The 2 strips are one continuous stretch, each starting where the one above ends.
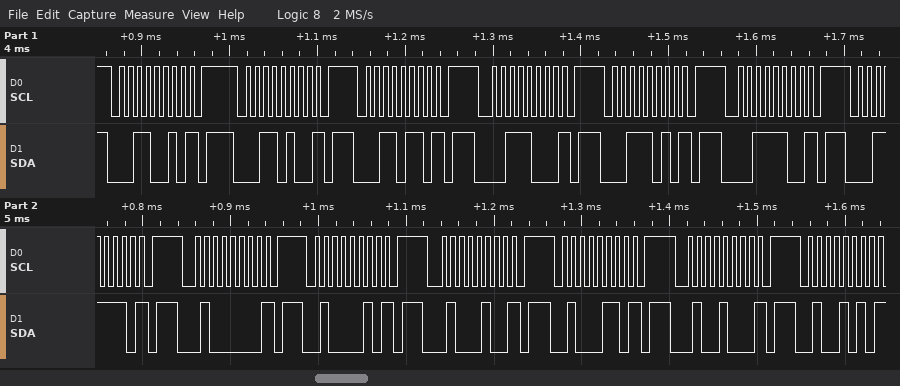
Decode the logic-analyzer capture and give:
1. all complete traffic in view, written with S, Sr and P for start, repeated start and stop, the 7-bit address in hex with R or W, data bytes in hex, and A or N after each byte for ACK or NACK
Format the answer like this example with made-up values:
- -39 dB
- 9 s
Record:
- S 19W N P S 1AW N P S 1BW N P S 1CW N P S 1DW N P S 1EW N P S 1FW N P S 20W N P S 21W N P S 22W N P S 23W N P S 24W N P S 25W N
